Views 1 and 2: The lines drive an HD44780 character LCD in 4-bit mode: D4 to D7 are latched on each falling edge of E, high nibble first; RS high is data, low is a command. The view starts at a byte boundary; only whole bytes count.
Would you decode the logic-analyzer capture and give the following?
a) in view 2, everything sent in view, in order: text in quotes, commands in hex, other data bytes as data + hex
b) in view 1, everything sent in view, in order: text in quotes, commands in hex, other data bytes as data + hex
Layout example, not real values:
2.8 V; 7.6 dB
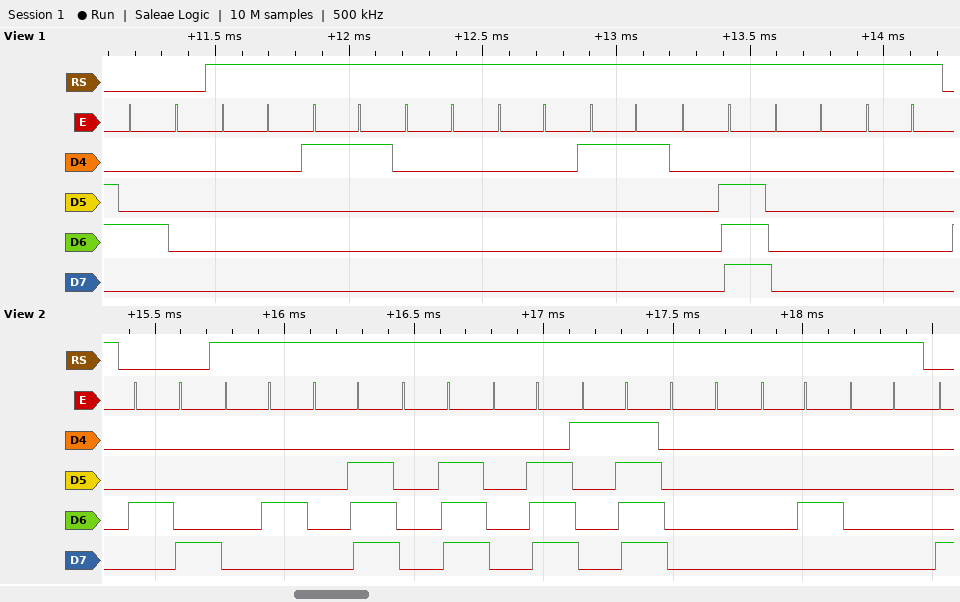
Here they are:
0x48 data 04 0E 0E 0E 1F 00 04 00; 0x40 data 00 11 00 00 11 0E 00 00
